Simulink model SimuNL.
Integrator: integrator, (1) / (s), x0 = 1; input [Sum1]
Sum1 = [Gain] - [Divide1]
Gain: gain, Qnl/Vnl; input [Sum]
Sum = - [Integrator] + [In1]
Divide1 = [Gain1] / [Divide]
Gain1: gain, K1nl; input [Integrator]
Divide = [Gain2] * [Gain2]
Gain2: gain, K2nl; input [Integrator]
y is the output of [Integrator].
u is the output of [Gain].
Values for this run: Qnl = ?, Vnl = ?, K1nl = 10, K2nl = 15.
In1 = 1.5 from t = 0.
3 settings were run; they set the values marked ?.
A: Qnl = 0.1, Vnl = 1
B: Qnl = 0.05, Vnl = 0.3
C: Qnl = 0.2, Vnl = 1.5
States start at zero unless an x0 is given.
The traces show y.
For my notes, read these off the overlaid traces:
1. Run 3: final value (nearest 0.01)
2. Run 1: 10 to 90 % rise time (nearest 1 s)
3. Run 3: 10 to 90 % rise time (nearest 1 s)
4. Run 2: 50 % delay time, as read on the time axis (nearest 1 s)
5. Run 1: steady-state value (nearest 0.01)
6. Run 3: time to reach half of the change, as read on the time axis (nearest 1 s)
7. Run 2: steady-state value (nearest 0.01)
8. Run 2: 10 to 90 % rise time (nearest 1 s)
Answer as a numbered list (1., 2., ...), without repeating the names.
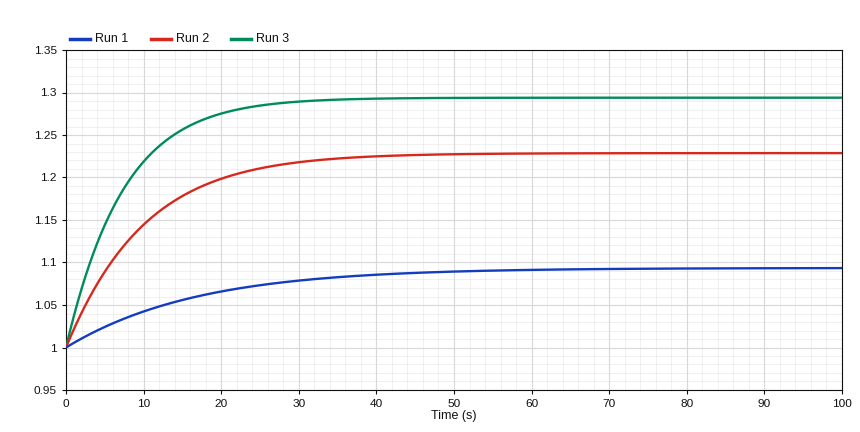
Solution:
1. 1.29
2. 36 s
3. 16 s
4. 7 s
5. 1.09
6. 5 s
7. 1.23
8. 22 s
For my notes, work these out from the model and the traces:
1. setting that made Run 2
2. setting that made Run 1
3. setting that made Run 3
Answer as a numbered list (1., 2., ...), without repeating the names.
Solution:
1. C
2. A
3. B
